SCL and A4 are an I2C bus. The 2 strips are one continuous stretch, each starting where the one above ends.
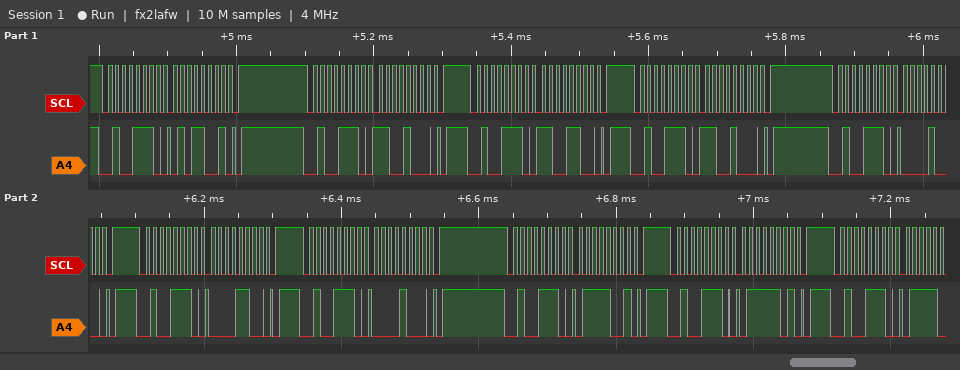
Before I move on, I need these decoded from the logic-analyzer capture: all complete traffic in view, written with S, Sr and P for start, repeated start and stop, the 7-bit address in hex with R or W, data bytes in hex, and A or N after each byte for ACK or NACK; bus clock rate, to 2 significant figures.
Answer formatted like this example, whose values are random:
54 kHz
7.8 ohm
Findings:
S 27W A 59 A P S 27W A C8 A P S 27W A CC A P S 27W A C8 A P S 27W A 08 A P S 27W A 0C A P S 27W A 08 A P S 27W A 79 A P S 27W A 7D A P S 27W A
100 kHz
